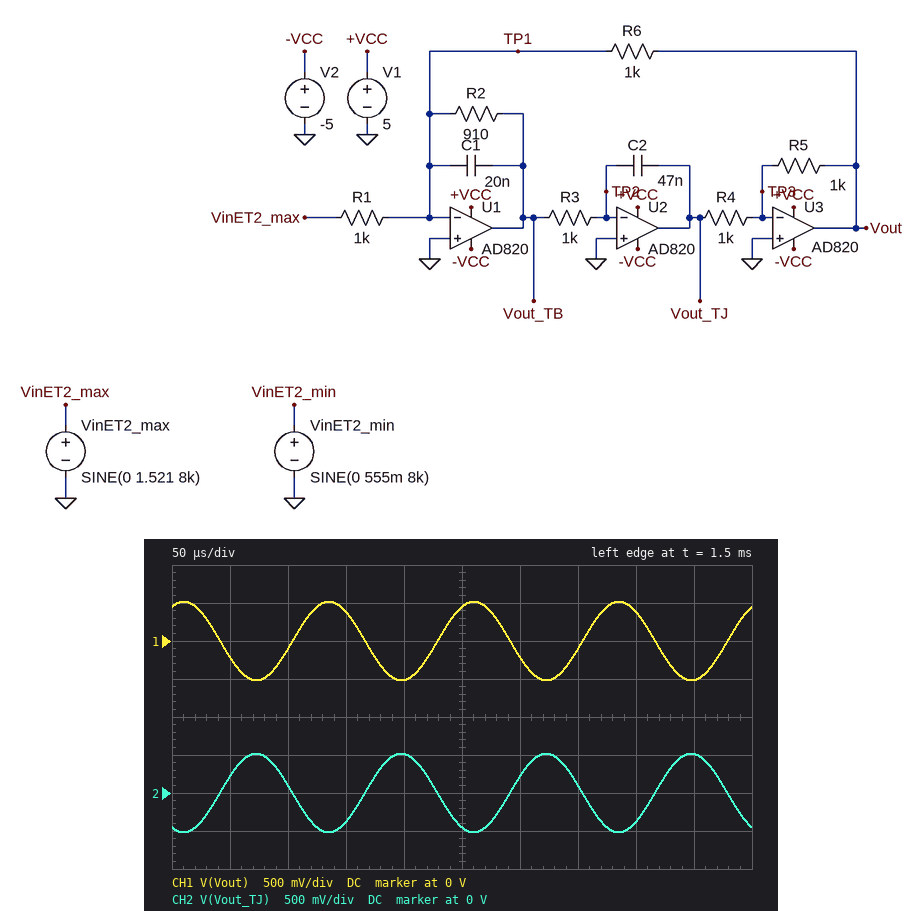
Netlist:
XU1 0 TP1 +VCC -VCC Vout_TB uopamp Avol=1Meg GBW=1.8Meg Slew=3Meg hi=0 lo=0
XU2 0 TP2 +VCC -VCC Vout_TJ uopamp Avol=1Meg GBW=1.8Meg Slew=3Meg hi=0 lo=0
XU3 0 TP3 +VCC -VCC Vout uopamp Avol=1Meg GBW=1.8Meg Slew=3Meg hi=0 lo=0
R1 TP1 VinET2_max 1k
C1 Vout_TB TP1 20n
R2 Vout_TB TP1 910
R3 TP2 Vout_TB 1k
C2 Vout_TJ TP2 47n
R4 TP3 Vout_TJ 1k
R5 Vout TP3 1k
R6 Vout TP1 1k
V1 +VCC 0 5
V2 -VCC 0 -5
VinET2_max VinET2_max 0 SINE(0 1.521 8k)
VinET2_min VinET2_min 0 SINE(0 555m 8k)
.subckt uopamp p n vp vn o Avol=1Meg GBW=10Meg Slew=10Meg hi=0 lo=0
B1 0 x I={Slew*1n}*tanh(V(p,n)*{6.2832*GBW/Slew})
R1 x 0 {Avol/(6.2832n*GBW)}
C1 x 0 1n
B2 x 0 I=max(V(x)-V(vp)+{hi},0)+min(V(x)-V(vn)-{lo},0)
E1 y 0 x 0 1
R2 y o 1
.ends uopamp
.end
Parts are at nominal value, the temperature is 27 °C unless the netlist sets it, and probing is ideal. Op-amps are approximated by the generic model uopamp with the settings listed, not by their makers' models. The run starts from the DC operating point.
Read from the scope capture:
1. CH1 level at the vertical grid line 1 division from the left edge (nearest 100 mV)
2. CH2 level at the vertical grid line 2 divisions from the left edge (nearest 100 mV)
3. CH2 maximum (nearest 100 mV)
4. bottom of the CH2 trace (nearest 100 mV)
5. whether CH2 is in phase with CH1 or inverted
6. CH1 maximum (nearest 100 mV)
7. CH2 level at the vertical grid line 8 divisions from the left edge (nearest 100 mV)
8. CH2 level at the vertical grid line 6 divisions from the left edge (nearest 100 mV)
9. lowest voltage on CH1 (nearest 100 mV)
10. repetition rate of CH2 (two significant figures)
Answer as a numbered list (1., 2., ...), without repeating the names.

1. -200 mV
2. 100 mV
3. 500 mV
4. -500 mV
5. inverted
6. 500 mV
7. -400 mV
8. 200 mV
9. -500 mV
10. 8.0 kHz
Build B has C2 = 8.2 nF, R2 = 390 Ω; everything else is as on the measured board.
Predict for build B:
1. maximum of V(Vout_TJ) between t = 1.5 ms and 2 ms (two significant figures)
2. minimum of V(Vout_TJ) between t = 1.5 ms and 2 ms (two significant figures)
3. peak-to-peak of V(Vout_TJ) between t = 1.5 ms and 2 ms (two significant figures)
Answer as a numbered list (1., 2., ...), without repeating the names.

1. 1.3 V
2. -1.3 V
3. 2.5 V
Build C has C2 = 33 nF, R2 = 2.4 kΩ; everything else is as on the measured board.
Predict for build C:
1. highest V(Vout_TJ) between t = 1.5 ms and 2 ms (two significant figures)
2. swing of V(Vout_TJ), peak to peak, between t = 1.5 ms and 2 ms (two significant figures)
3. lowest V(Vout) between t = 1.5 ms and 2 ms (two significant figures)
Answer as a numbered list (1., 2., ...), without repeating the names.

1. 1.6 V
2. 3.2 V
3. -1.6 V
